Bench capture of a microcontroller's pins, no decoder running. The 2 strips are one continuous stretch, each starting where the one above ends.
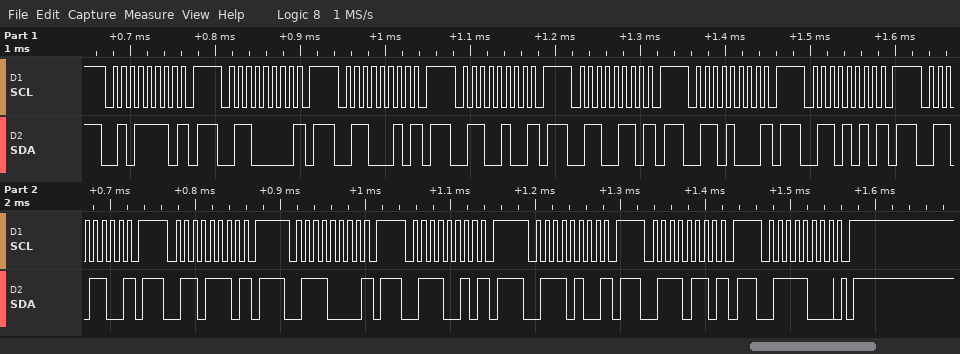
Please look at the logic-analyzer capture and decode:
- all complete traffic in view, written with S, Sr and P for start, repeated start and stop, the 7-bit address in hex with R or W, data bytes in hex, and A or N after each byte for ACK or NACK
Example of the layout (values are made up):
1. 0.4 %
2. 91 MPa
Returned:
1. S 2FW N P S 30W N P S 31W N P S 32W N P S 33W N P S 34W N P S 35W N P S 36W N P S 37W N P S 38W N P S 39W N P S 3AW N P S 3BW N P S 3CW A P
